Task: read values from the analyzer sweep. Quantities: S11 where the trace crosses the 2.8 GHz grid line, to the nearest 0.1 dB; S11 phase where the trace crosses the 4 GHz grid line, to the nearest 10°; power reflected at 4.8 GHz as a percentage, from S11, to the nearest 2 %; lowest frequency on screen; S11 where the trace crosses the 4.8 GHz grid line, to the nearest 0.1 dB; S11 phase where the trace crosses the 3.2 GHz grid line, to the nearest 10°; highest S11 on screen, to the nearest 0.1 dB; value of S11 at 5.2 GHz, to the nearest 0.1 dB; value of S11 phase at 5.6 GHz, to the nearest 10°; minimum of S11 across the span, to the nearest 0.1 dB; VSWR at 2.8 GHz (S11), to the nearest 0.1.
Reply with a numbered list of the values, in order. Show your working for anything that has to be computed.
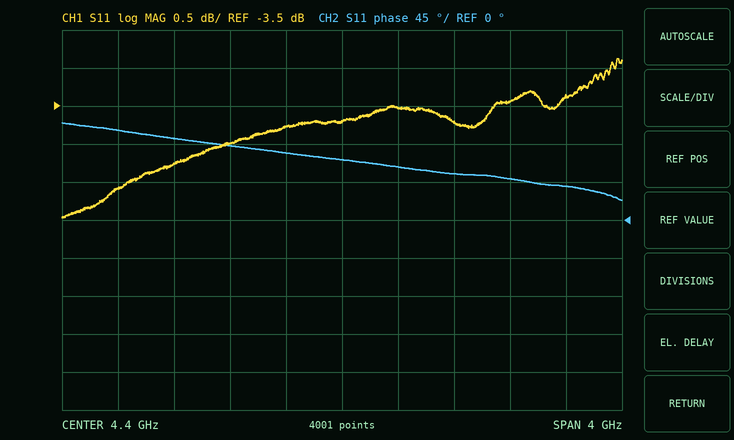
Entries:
1. -4.6 dB
2. 80°
3. 10^(-3.5/10) ≈ 44.7 %, so 44 % to the nearest 2 %
4. 2.4 GHz
5. -3.5 dB
6. 100°
7. -2.9 dB
8. -3.7 dB
9. 50°
10. -5.0 dB
11. |Γ| = 10^(-4.6/20) = 0.5888; VSWR = (1 + 0.5888)/(1 − 0.5888) ≈ 3.9
